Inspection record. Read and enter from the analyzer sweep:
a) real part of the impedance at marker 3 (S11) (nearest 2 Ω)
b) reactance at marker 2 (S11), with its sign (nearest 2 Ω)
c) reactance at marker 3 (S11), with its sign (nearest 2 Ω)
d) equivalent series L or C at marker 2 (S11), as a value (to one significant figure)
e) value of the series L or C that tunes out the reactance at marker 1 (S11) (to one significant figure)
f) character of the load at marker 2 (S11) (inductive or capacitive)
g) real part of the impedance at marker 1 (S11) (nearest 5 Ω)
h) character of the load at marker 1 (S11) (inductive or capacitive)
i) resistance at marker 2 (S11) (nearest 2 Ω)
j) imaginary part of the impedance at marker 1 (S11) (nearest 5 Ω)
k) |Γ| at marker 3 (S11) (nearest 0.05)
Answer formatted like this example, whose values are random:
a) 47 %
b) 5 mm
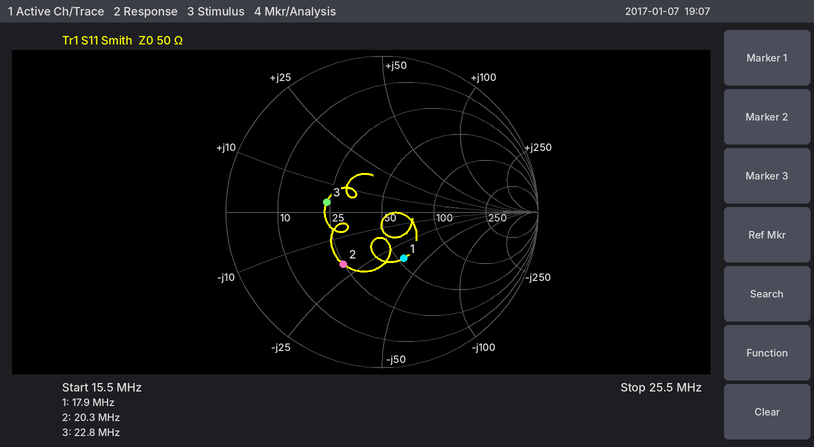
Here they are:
a) 24 Ω
b) -20 Ω
c) +4 Ω
d) 400 pF
e) 300 nH
f) capacitive
g) 55 Ω
h) capacitive
i) 24 Ω
j) -35 Ω
k) 0.35
